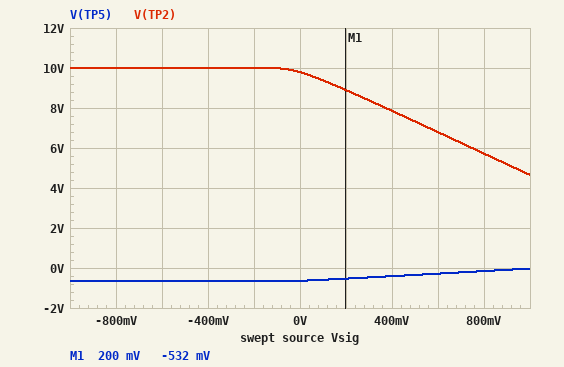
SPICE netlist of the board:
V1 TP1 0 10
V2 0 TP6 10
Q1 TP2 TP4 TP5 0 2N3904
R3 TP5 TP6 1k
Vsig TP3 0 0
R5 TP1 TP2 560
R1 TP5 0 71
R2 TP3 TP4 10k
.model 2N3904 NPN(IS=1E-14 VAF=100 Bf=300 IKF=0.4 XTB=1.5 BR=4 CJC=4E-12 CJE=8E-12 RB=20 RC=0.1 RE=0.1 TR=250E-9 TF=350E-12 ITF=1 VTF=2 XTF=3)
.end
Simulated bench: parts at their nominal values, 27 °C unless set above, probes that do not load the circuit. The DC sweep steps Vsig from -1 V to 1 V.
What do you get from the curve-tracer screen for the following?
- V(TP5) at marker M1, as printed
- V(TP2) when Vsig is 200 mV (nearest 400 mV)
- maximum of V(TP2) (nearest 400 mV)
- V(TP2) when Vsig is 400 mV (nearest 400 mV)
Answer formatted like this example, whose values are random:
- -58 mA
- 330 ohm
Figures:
- -532 mV
- 8.8 V
- 10.0 V
- 8.0 V
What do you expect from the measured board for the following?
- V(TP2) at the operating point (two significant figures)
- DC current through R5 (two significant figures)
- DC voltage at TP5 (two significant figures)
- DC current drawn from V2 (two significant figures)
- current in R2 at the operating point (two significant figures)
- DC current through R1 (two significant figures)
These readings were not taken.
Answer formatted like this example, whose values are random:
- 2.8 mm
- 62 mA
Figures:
- 9.8 V
- 370 µA
- -640 mV
- 9.4 mA
- 1.1 µA
- 9.0 mA
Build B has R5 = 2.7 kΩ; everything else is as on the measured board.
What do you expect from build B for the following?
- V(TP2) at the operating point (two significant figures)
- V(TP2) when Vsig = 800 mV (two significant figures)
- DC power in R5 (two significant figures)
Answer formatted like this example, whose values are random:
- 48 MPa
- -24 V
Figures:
- 9.0 V
- -320 mV
- 370 µW
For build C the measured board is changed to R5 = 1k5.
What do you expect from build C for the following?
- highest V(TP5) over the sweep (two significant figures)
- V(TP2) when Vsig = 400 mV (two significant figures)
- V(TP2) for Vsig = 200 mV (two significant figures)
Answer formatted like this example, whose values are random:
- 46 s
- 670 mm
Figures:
- -210 mV
- 4.3 V
- 7.1 V
